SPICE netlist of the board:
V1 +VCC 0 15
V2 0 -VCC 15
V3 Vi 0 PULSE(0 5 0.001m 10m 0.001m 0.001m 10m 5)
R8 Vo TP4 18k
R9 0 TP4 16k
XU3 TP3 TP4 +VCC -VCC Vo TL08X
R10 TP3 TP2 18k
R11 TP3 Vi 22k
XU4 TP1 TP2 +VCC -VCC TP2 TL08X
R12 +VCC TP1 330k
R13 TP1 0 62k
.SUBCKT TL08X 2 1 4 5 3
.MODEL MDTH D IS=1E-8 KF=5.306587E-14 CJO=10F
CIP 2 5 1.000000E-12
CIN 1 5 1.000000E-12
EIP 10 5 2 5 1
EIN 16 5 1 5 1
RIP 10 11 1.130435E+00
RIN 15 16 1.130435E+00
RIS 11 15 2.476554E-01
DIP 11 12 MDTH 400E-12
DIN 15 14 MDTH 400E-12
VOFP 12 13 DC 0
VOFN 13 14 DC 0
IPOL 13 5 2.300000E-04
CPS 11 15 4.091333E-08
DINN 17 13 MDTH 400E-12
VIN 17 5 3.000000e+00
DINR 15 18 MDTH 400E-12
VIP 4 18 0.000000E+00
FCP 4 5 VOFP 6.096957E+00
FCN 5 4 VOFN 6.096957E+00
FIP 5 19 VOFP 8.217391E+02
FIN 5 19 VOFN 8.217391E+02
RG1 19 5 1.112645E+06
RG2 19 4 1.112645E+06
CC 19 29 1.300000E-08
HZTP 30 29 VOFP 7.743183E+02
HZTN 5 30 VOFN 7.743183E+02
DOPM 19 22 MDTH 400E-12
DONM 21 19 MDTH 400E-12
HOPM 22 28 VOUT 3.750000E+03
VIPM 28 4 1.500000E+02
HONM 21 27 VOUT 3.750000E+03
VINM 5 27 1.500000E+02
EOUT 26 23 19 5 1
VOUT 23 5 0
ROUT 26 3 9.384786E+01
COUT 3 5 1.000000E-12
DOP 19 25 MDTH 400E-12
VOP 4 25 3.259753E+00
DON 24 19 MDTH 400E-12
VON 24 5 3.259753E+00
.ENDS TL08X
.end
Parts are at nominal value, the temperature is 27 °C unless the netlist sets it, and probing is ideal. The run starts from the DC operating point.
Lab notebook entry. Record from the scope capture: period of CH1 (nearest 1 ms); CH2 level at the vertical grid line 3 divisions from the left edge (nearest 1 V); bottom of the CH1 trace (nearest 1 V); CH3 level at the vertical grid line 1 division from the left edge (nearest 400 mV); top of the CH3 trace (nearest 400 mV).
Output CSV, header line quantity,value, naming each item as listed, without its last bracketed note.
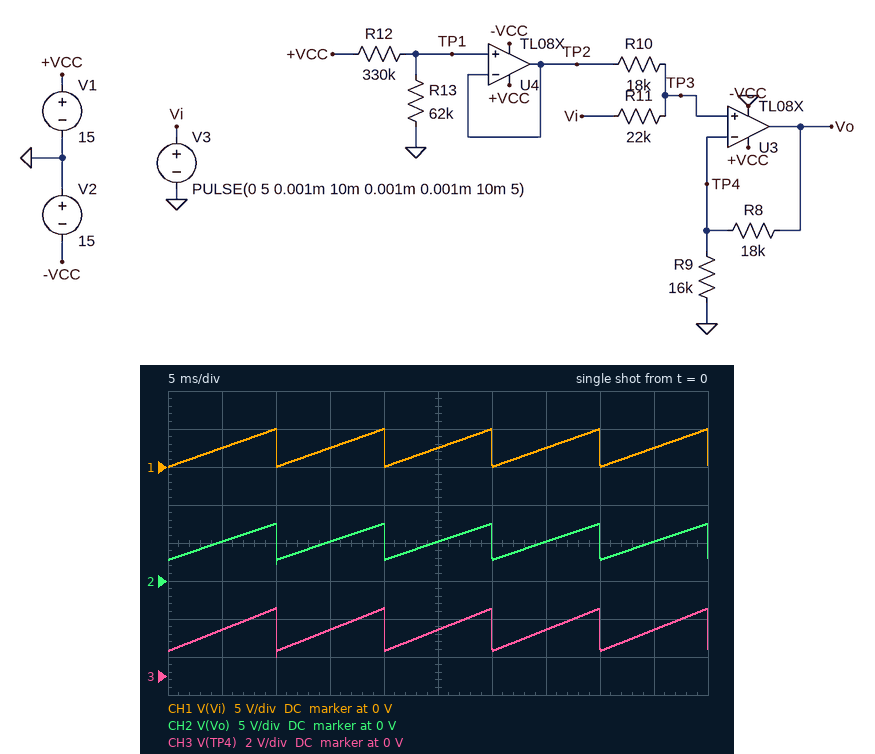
quantity,value
period of CH1,10 ms
CH2 level at the vertical grid line 3 divisions from the left edge,5 V
bottom of the CH1 trace,0 V
CH3 level at the vertical grid line 1 division from the left edge,2.4 V
top of the CH3 trace,3.6 V
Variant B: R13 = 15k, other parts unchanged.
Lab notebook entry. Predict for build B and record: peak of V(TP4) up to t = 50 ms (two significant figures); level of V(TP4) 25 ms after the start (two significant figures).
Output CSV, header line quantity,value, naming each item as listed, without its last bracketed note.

quantity,value
peak of V(TP4) up to t = 50 ms,2.6 V
level of V(TP4) 25 ms after the start,1.5 V
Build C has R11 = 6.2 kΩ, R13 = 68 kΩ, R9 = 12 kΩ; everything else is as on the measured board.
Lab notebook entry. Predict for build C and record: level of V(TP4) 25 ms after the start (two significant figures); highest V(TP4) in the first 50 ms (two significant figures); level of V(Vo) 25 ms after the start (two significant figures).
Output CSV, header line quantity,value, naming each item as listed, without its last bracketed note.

quantity,value
level of V(TP4) 25 ms after the start,2.5 V
highest V(TP4) in the first 50 ms,4.4 V
level of V(Vo) 25 ms after the start,6.3 V
